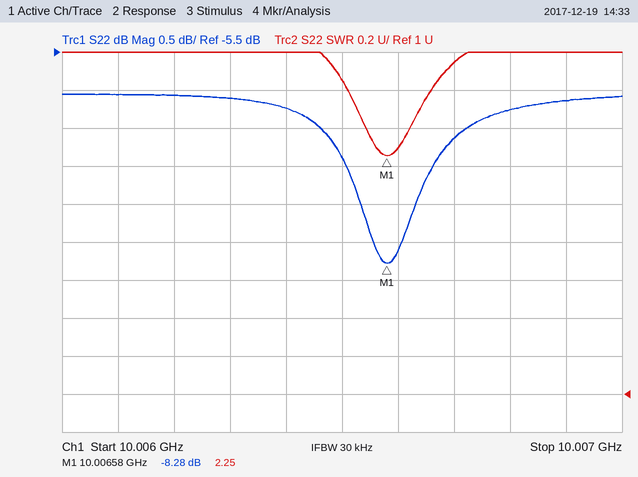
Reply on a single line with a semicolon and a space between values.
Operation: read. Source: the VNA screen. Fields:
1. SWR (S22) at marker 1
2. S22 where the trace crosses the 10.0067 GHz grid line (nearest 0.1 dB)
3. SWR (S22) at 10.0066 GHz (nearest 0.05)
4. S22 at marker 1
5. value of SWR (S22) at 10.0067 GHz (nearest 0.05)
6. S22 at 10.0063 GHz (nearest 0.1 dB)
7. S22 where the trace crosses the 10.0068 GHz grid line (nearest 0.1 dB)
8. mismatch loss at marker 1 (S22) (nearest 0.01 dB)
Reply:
2.25; -6.6 dB; 2.30; -8.28 dB; 2.75; -6.1 dB; -6.3 dB; 0.70 dB
